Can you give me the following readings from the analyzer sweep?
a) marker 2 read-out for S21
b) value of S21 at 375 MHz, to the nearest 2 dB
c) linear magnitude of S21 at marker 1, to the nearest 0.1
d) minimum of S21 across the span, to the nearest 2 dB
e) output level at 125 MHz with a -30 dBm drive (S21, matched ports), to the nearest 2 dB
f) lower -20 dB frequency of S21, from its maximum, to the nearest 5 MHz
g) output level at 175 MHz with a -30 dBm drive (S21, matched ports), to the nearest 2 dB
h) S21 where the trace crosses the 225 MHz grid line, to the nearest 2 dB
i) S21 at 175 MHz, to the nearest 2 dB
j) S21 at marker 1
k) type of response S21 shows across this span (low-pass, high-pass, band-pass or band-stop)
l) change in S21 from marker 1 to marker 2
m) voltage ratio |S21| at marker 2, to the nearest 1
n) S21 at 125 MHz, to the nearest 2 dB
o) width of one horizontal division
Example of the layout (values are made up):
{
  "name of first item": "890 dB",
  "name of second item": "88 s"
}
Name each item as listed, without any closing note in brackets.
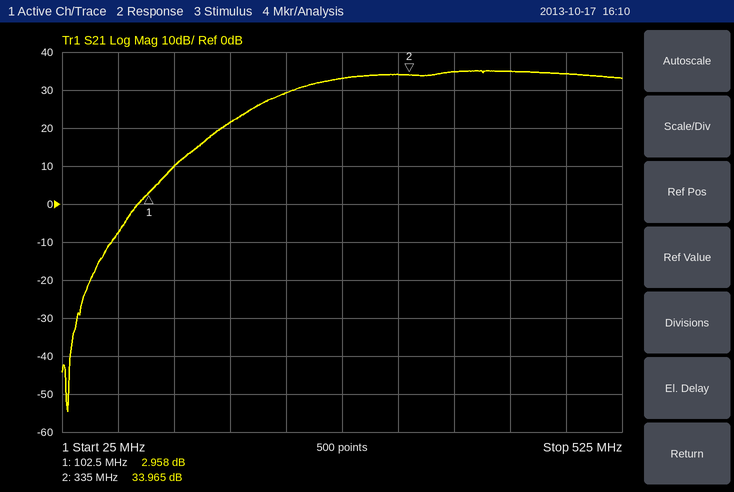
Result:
{
  "marker 2 read-out for S21": "33.965 dB",
  "value of S21 at 375 MHz, to the nearest 2 dB": "34 dB",
  "linear magnitude of S21 at marker 1, to the nearest 0.1": "1.4",
  "minimum of S21 across the span, to the nearest 2 dB": "-54 dB",
  "output level at 125 MHz with a -30 dBm drive (S21, matched ports), to the nearest 2 dB": "-20 dBm",
  "lower -20 dB frequency of S21, from its maximum, to the nearest 5 MHz": "145 MHz",
  "output level at 175 MHz with a -30 dBm drive (S21, matched ports), to the nearest 2 dB": "-8 dBm",
  "S21 where the trace crosses the 225 MHz grid line, to the nearest 2 dB": "30 dB",
  "S21 at 175 MHz, to the nearest 2 dB": "22 dB",
  "S21 at marker 1": "2.958 dB",
  "type of response S21 shows across this span": "high-pass",
  "change in S21 from marker 1 to marker 2": "31.007 dB",
  "voltage ratio |S21| at marker 2, to the nearest 1": "50",
  "S21 at 125 MHz, to the nearest 2 dB": "10 dB",
  "width of one horizontal division": "50 MHz"
}
